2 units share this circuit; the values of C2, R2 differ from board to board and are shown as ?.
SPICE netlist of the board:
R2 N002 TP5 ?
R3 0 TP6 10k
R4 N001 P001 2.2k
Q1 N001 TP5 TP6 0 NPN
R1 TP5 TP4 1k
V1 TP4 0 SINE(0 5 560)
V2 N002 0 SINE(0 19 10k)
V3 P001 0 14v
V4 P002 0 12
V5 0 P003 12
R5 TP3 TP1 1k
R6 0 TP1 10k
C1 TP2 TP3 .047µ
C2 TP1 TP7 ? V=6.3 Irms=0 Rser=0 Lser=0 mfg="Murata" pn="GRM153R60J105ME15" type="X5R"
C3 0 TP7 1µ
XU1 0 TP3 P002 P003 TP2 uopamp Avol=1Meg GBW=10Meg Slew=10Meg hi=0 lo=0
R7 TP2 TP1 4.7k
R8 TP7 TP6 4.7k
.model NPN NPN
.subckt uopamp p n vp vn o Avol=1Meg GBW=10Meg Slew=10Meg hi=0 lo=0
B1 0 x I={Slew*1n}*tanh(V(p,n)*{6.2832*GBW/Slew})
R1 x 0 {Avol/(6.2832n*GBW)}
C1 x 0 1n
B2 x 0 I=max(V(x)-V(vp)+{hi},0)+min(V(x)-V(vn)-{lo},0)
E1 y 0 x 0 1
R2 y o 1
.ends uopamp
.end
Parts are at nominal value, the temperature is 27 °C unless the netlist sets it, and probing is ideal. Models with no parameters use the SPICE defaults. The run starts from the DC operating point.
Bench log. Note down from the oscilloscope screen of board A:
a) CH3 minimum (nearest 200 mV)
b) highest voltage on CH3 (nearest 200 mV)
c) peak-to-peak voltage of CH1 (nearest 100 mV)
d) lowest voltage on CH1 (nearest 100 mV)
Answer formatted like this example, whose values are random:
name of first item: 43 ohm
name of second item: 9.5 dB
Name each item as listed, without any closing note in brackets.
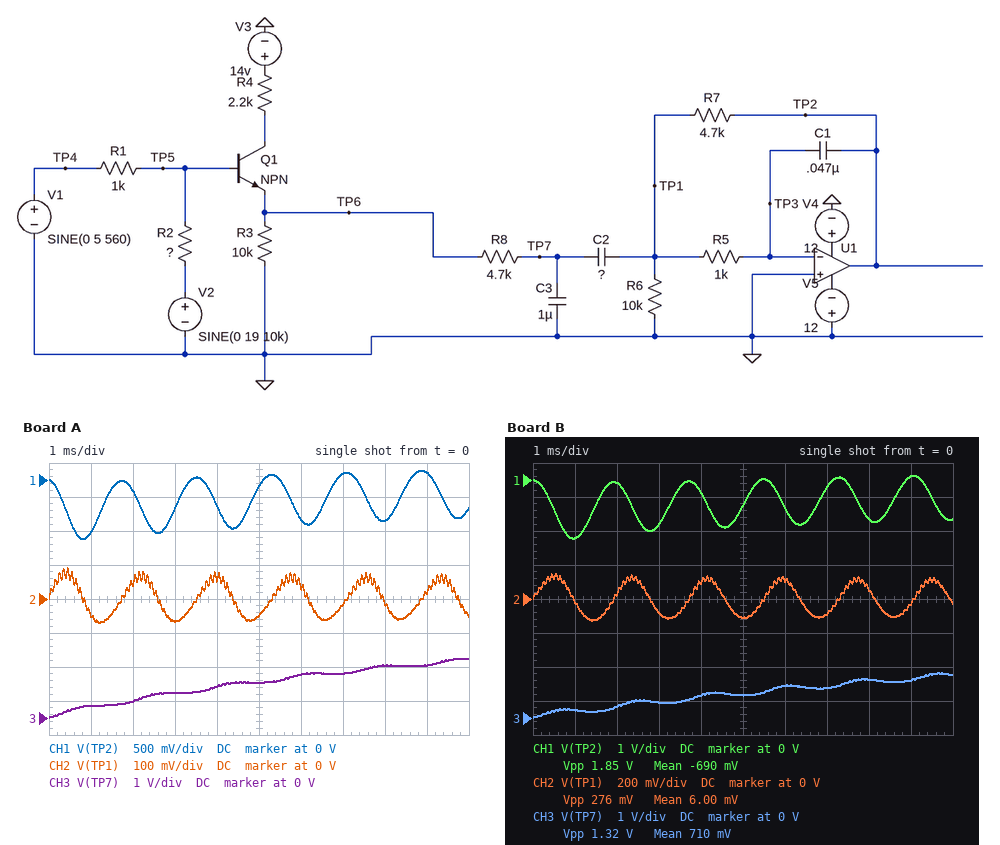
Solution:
CH3 minimum: 0 V
highest voltage on CH3: 1.8 V
peak-to-peak voltage of CH1: 1.0 V
lowest voltage on CH1: -900 mV
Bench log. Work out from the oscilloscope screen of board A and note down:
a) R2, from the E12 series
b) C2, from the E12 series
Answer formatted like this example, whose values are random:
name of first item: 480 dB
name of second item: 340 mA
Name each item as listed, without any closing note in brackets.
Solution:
R2, from the E12 series: 2.2 kΩ
C2, from the E12 series: 390 nF
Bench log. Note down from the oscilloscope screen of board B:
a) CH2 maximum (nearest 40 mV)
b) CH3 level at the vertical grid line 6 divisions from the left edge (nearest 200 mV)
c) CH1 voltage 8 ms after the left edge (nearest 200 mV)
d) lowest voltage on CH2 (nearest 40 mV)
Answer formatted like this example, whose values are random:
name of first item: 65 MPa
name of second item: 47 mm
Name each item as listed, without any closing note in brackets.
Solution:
CH2 maximum: 160 mV
CH3 level at the vertical grid line 6 divisions from the left edge: 1.0 V
CH1 voltage 8 ms after the left edge: -1.2 V
lowest voltage on CH2: -120 mV
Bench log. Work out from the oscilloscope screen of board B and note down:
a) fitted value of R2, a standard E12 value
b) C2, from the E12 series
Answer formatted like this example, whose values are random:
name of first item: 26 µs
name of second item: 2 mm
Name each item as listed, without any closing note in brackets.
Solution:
fitted value of R2, a standard E12 value: 2.2 kΩ
C2, from the E12 series: 1.2 µF
